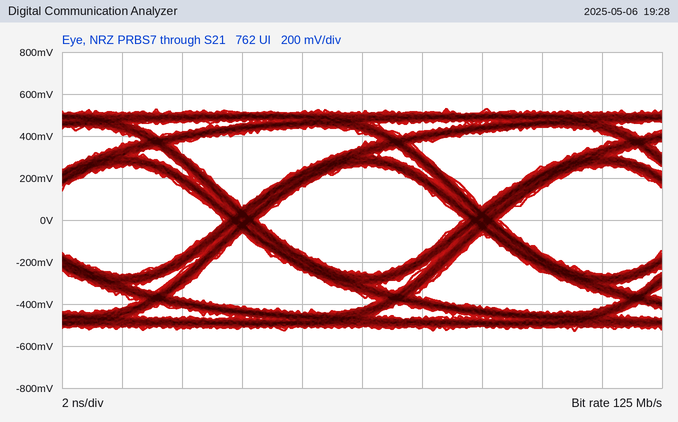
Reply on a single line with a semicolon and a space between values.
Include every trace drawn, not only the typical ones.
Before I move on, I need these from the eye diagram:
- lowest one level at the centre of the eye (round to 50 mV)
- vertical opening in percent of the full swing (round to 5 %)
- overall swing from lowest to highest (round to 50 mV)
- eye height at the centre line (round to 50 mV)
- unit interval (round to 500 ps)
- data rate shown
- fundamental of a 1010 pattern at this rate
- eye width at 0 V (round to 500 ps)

250 mV; 50 %; 1.05 V; 500 mV; 8.0 ns; 125 Mb/s; 62.5 MHz; 7.0 ns
